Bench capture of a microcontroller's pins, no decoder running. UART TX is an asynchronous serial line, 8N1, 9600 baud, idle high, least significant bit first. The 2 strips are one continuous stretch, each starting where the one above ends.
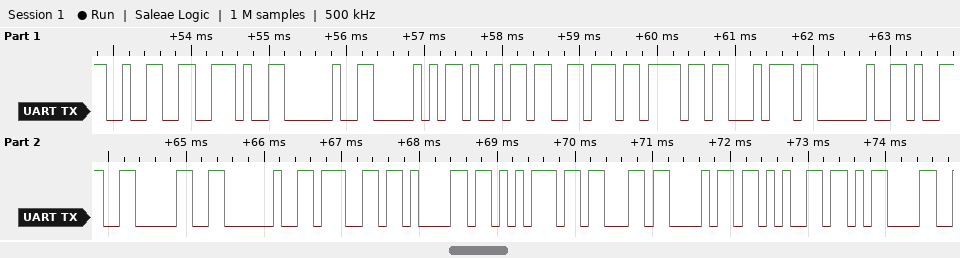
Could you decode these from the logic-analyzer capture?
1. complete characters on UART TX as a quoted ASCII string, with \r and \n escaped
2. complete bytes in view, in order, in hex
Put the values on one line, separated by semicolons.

"2. Pivot 90 gauche\r"; 0x32 0x2E 0x20 0x50 0x69 0x76 0x6F 0x74 0x20 0x39 0x30 0x20 0x67 0x61 0x75 0x63 0x68 0x65 0x0D
